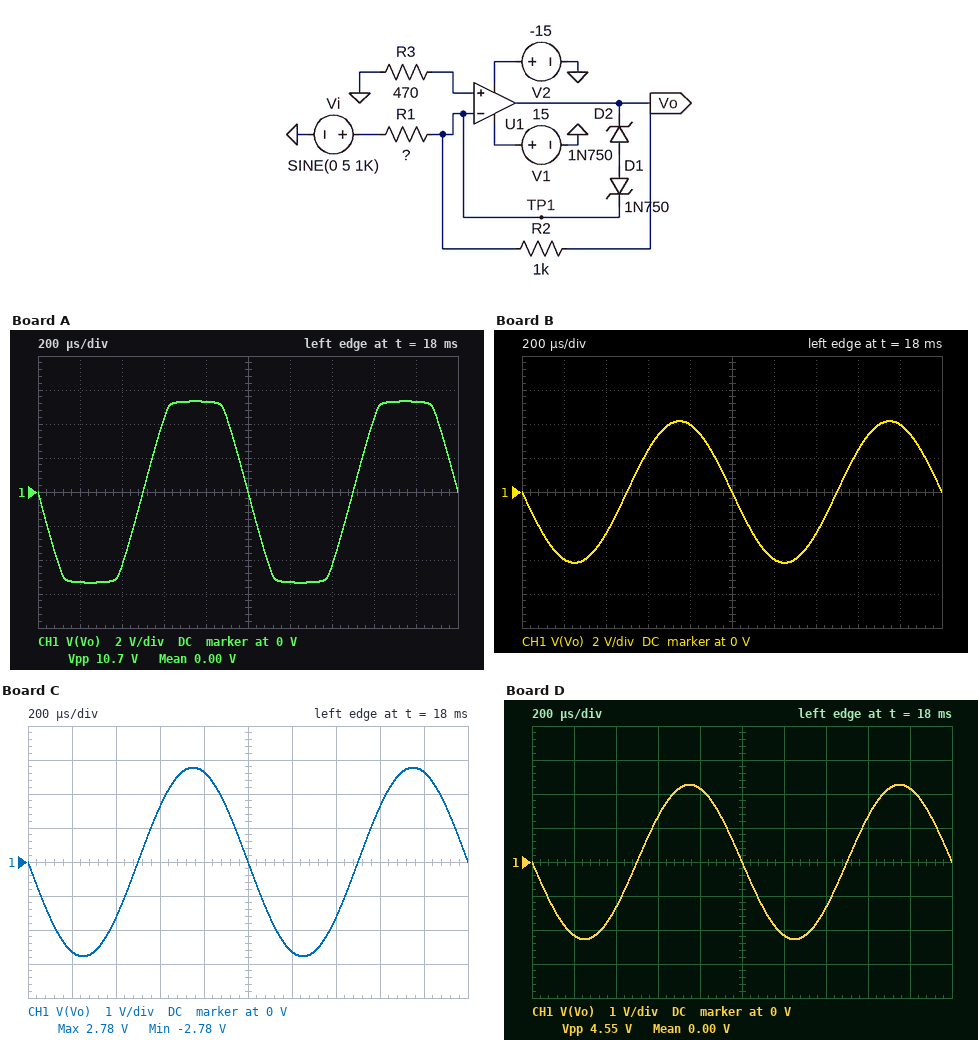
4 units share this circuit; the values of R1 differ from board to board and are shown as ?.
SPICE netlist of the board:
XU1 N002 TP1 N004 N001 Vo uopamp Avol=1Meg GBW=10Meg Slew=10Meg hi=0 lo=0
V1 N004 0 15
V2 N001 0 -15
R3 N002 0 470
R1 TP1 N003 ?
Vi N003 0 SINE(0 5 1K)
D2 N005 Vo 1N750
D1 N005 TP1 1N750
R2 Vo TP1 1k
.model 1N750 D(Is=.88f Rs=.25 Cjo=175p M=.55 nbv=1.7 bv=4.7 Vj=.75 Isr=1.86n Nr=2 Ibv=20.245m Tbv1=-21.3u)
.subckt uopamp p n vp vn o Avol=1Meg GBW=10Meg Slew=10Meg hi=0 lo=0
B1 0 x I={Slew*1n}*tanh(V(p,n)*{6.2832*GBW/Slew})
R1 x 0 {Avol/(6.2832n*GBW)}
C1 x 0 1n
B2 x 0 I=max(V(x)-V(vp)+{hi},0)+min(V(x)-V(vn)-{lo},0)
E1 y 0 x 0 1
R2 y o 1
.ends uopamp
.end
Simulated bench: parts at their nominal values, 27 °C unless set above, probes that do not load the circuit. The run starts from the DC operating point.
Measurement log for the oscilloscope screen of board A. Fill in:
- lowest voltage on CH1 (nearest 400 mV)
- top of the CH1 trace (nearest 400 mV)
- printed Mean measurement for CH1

-5.2 V
5.2 V
0.00 V
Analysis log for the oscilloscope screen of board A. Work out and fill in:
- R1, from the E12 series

680 Ω
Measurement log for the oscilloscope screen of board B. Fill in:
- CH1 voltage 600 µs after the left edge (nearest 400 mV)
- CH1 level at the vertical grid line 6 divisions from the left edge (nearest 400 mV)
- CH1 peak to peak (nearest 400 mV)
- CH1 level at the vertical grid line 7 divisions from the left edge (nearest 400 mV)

2.4 V
-4.0 V
8.4 V
-2.4 V
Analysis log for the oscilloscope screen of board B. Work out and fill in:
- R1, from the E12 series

1.2 kΩ
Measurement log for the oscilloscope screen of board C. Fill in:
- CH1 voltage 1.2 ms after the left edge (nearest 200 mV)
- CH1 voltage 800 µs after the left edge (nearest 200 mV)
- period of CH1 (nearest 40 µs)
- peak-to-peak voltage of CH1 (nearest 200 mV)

-2.6 V
2.6 V
1.00 ms
5.6 V
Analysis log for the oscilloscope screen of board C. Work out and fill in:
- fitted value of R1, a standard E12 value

1.8 kΩ
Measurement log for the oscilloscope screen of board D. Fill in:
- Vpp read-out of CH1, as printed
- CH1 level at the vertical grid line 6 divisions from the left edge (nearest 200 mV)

4.55 V
-2.2 V
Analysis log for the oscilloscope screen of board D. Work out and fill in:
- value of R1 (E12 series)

2.2 kΩ
